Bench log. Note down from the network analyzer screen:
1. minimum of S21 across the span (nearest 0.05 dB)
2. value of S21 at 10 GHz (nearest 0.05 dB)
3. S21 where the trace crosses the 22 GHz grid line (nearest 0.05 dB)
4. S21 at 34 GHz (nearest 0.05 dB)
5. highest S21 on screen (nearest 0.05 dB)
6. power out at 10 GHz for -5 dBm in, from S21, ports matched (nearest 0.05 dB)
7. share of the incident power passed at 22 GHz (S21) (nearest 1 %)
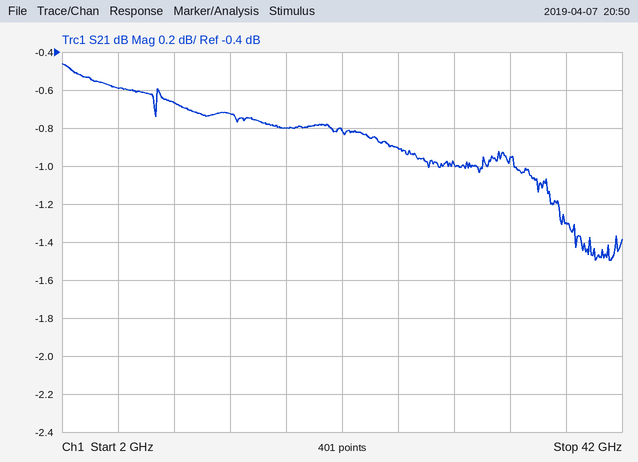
-1.50 dB
-0.65 dB
-0.80 dB
-0.95 dB
-0.45 dB
-5.65 dBm
83 %
